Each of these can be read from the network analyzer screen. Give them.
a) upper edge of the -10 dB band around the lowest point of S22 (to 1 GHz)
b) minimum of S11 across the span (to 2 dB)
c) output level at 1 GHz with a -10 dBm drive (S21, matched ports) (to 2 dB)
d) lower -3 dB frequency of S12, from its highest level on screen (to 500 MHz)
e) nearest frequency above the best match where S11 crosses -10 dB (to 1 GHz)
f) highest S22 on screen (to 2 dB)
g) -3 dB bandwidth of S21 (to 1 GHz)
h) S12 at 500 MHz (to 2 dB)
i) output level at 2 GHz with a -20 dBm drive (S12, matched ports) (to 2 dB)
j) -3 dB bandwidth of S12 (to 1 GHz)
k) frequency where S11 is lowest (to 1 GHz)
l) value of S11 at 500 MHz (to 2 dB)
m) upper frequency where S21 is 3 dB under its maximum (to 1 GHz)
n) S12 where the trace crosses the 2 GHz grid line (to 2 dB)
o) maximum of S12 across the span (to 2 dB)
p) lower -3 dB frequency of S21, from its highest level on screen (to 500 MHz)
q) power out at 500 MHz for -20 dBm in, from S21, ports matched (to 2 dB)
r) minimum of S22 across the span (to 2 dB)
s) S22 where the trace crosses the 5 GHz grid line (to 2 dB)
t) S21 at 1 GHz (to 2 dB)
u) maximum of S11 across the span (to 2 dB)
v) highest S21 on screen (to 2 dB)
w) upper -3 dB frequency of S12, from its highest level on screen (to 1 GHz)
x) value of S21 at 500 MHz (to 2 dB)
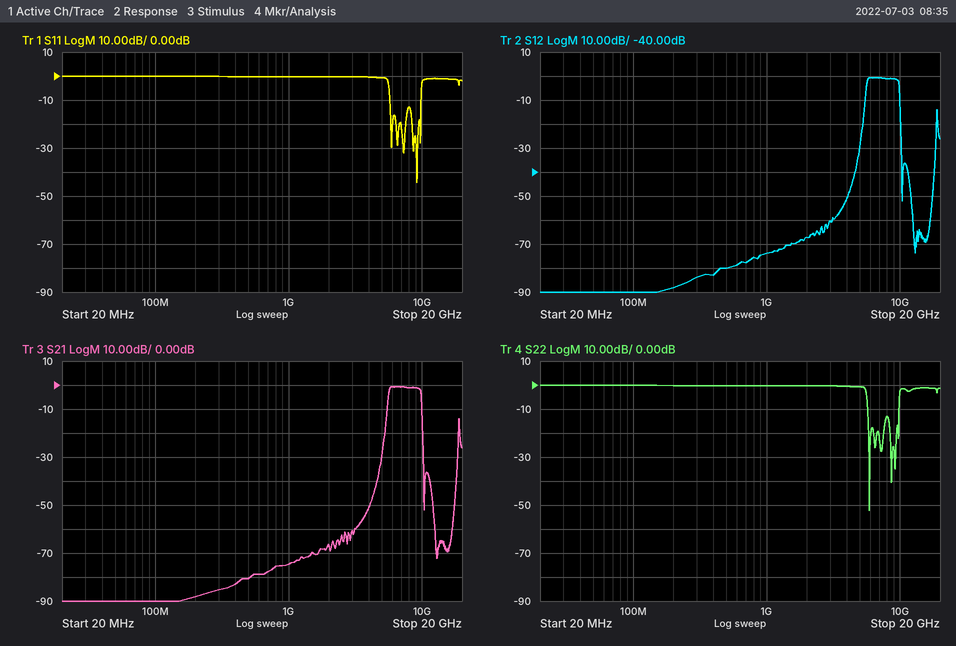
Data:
10 GHz
-44 dB
-84 dBm
5.5 GHz
10 GHz
0 dB
4 GHz
-80 dB
-88 dBm
4 GHz
9 GHz
0 dB
10 GHz
-68 dB
0 dB
5.5 GHz
-100 dBm
-52 dB
0 dB
-74 dB
0 dB
0 dB
10 GHz
-80 dB
